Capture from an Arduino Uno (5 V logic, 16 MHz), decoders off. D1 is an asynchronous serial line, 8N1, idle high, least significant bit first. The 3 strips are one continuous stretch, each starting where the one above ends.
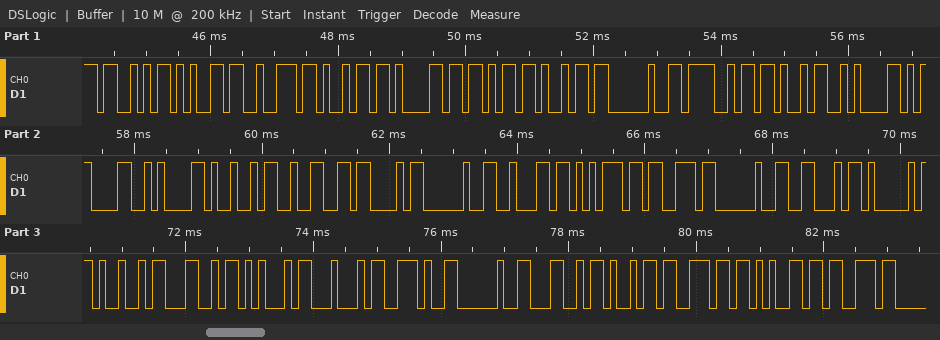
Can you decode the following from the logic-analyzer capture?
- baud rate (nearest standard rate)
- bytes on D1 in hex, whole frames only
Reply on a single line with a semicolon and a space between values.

9600 baud; 0x53 0x65 0x72 0x69 0x61 0x6B 0x69 0x20 0x4F 0x4B 0x0A 0x0D 0x0A 0x49 0x32 0x43 0x20 0x62 0x75 0x73 0x20 0x46 0x41 0x49 0x4C 0x45 0x44 0x2E 0x20 0x4C 0x69 0x6E 0x65 0x73
